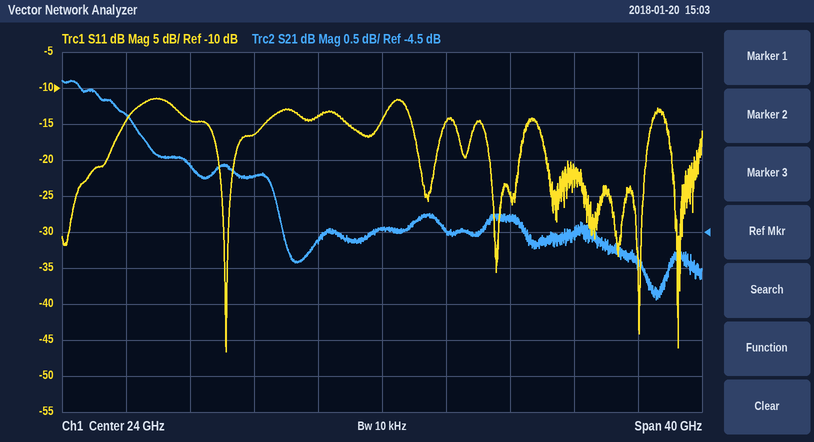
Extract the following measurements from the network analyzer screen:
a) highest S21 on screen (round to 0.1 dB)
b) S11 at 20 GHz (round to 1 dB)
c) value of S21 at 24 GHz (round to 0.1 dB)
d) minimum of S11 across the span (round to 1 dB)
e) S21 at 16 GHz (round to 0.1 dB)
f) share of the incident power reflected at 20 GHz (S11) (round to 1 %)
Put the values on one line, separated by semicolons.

-2.4 dB; -14 dB; -4.5 dB; -47 dB; -3.7 dB; 4 %
